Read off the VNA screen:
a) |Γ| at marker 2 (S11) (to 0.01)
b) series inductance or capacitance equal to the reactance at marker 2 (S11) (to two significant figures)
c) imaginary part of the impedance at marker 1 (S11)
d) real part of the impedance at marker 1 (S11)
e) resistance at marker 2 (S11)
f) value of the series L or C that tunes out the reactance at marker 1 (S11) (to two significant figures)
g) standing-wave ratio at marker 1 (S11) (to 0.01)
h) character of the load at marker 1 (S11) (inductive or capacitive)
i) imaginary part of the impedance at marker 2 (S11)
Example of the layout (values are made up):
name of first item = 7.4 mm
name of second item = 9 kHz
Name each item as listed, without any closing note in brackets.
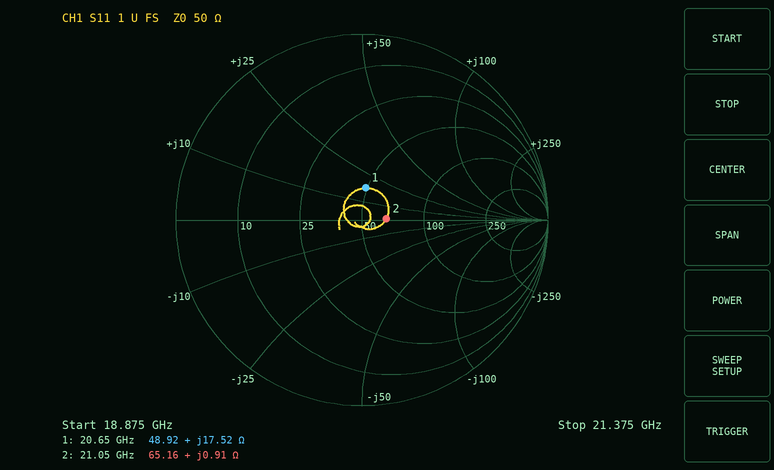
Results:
|Γ| at marker 2 (S11) = 0.13
series inductance or capacitance equal to the reactance at marker 2 (S11) = 6.9 pH
imaginary part of the impedance at marker 1 = +17.52 Ω
real part of the impedance at marker 1 = 48.92 Ω
resistance at marker 2 = 65.16 Ω
value of the series L or C that tunes out the reactance at marker 1 (S11) = 440 fF
standing-wave ratio at marker 1 (S11) = 1.42
character of the load at marker 1 (S11) = inductive
imaginary part of the impedance at marker 2 = +0.91 Ω
